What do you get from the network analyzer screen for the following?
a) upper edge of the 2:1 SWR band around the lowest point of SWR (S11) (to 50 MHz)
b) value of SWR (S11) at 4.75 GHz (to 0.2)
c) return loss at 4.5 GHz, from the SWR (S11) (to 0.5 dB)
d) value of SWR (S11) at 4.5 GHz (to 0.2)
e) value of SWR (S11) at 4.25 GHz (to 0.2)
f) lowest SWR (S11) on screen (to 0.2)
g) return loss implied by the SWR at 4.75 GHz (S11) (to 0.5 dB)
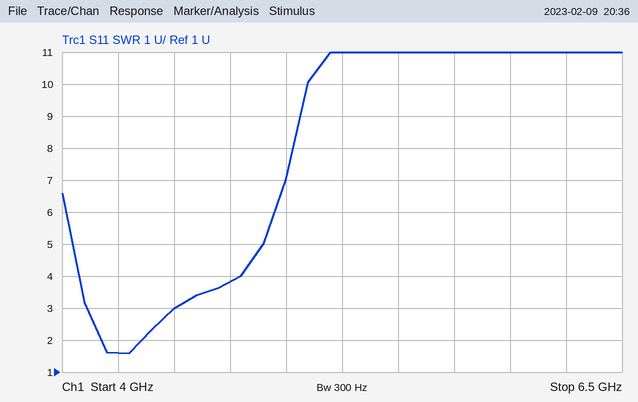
4.35 GHz
3.8
6.0 dB
3.0
1.6
1.6
4.5 dB
